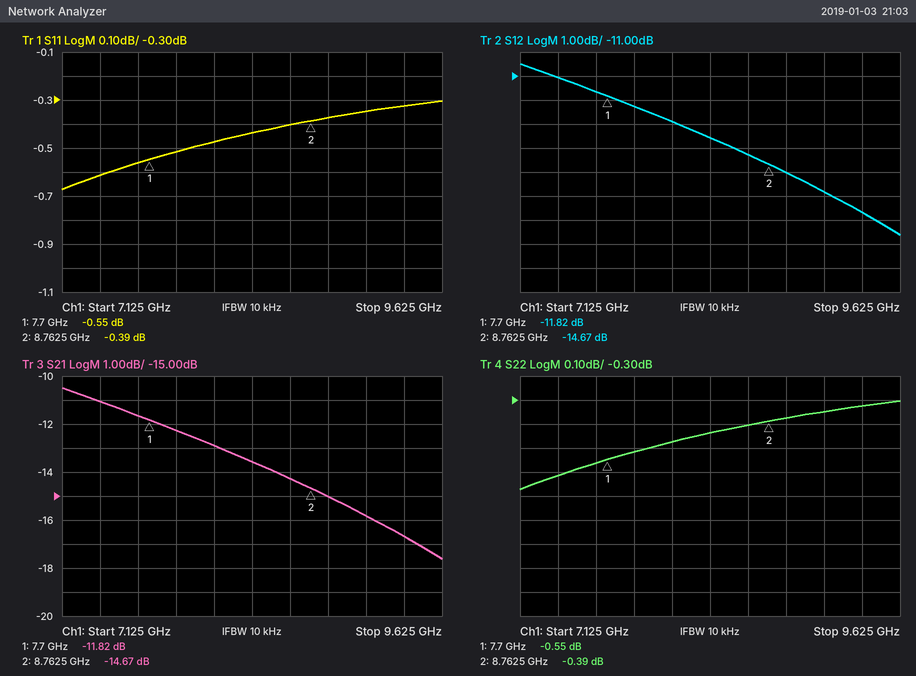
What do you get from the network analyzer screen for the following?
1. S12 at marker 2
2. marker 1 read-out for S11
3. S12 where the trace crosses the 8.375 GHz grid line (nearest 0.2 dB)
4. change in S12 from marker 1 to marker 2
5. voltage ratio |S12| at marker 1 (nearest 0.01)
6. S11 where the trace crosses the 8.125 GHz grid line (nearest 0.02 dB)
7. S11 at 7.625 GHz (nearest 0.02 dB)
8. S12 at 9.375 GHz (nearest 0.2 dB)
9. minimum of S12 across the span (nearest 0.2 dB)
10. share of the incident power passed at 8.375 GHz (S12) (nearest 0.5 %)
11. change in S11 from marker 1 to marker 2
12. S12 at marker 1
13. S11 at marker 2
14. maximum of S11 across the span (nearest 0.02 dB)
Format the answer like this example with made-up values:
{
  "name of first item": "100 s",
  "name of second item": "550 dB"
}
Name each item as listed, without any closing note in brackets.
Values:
{
  "S12 at marker 2": "-14.67 dB",
  "marker 1 read-out for S11": "-0.55 dB",
  "S12 where the trace crosses the 8.375 GHz grid line": "-13.6 dB",
  "change in S12 from marker 1 to marker 2": "-2.85 dB",
  "voltage ratio |S12| at marker 1": "0.26",
  "S11 where the trace crosses the 8.125 GHz grid line": "-0.48 dB",
  "S11 at 7.625 GHz": "-0.56 dB",
  "S12 at 9.375 GHz": "-16.6 dB",
  "minimum of S12 across the span": "-17.6 dB",
  "share of the incident power passed at 8.375 GHz (S12)": "4.5 %",
  "change in S11 from marker 1 to marker 2": "0.16 dB",
  "S12 at marker 1": "-11.82 dB",
  "S11 at marker 2": "-0.39 dB",
  "maximum of S11 across the span": "-0.30 dB"
}
